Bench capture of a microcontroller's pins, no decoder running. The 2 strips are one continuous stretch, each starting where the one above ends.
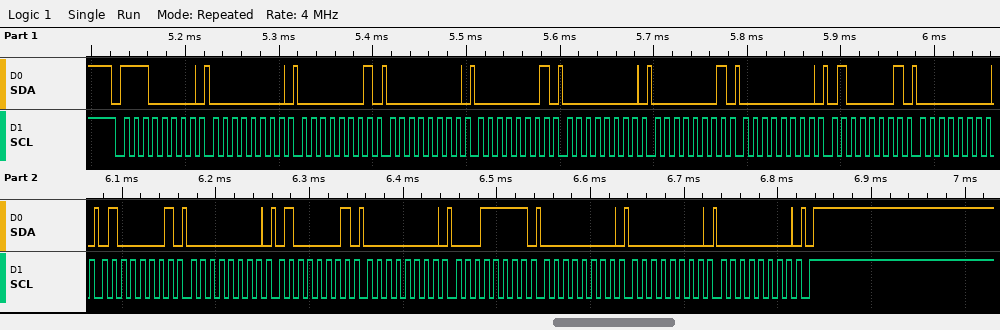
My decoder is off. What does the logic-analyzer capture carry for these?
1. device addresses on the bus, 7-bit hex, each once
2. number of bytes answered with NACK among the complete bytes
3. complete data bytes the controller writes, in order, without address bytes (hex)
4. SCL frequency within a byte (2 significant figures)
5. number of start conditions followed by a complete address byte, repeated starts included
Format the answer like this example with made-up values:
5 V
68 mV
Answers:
0x70
0
00 01 00 01 00 01 00 41 00 41 00 41 00 1F 00 00 00
100 kHz
1
